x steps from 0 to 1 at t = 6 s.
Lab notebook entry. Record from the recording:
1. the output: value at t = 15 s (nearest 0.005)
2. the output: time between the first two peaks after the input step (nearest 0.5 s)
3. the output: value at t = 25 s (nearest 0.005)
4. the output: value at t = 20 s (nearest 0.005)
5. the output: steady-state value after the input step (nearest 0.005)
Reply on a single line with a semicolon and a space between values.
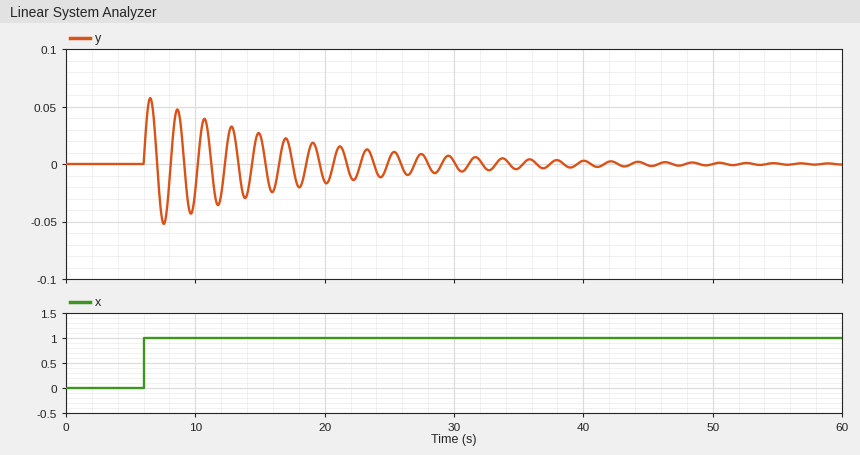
0.025; 2.0 s; 0.005; -0.015; 0.000
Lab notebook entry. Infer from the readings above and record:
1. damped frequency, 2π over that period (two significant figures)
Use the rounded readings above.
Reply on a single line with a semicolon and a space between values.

3.1 rad/s
